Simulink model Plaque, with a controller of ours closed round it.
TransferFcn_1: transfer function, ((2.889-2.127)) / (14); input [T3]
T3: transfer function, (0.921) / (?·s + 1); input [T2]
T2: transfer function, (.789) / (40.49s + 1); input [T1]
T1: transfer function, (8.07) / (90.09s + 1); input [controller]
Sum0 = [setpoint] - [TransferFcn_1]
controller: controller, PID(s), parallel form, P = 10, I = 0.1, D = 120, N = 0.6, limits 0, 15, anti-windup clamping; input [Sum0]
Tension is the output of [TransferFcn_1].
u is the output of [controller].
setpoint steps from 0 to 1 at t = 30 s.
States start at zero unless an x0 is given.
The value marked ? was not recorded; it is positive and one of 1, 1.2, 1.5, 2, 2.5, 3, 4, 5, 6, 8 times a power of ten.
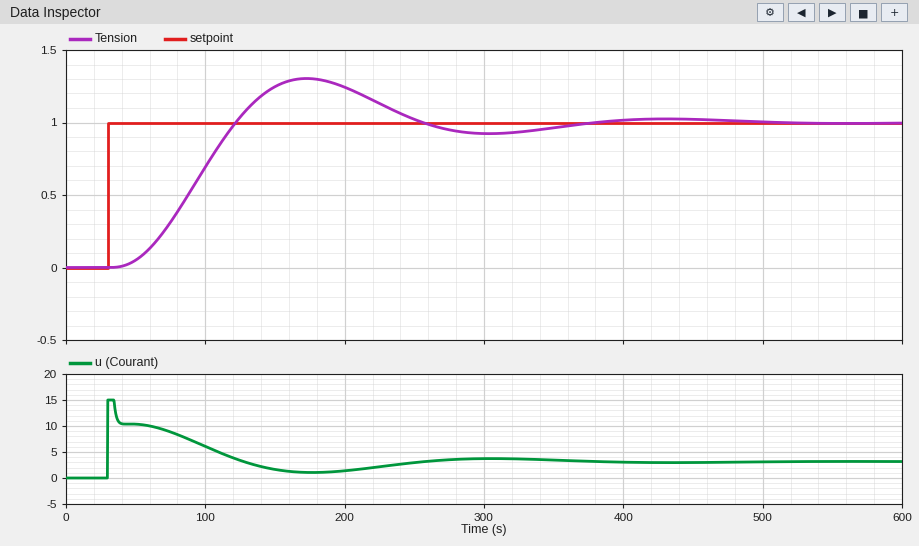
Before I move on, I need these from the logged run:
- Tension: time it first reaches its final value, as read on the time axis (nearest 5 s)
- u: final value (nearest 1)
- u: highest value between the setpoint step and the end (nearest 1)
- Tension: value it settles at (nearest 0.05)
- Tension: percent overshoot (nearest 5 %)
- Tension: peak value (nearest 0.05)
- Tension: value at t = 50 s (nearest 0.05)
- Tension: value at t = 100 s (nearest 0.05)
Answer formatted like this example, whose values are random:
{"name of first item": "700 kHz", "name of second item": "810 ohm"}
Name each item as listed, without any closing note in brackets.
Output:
{"Tension: time it first reaches its final value, as read on the time axis": "120 s", "u: final value": "3", "u: highest value between the setpoint step and the end": "15", "Tension: value it settles at": "1.00", "Tension: percent overshoot": "30 %", "Tension: peak value": "1.30", "Tension: value at t = 50 s": "0.05", "Tension: value at t = 100 s": "0.70"}
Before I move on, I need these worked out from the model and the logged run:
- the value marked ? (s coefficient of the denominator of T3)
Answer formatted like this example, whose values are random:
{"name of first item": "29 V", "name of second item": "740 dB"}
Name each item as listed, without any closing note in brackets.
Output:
{"the value marked ?": "20"}
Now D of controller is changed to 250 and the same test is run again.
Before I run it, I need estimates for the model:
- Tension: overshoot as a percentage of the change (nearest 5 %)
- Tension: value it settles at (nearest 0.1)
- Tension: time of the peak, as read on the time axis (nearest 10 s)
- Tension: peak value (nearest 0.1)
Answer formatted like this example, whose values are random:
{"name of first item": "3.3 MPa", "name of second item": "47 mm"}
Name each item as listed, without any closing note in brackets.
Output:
{"Tension: overshoot as a percentage of the change": "20 %", "Tension: value it settles at": "1.0", "Tension: time of the peak, as read on the time axis": "190 s", "Tension: peak value": "1.2"}
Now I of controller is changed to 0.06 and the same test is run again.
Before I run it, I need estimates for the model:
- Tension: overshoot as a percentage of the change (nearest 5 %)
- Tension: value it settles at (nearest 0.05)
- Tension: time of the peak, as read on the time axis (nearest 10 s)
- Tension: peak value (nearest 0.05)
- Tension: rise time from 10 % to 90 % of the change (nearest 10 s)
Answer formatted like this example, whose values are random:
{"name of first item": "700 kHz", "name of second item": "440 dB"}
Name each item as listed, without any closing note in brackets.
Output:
{"Tension: overshoot as a percentage of the change": "15 %", "Tension: value it settles at": "1.00", "Tension: time of the peak, as read on the time axis": "170 s", "Tension: peak value": "1.15", "Tension: rise time from 10 % to 90 % of the change": "60 s"}
